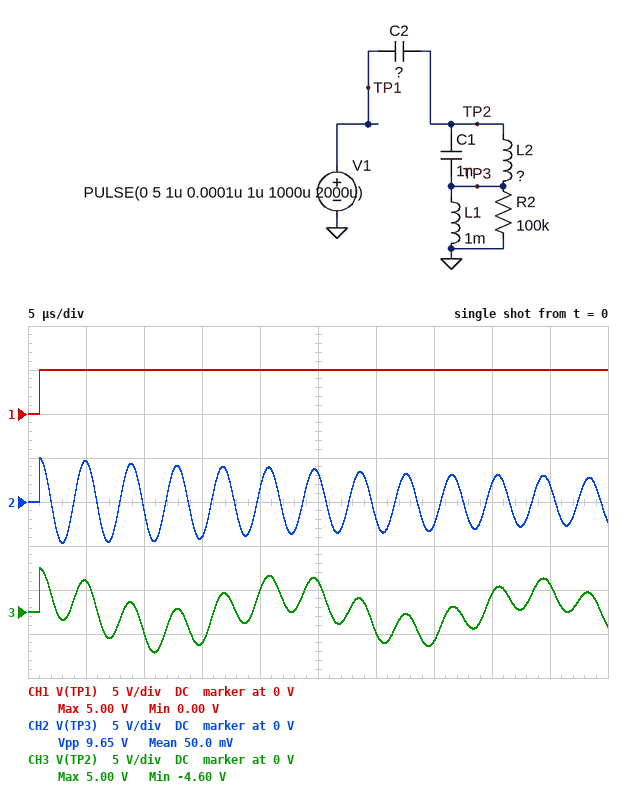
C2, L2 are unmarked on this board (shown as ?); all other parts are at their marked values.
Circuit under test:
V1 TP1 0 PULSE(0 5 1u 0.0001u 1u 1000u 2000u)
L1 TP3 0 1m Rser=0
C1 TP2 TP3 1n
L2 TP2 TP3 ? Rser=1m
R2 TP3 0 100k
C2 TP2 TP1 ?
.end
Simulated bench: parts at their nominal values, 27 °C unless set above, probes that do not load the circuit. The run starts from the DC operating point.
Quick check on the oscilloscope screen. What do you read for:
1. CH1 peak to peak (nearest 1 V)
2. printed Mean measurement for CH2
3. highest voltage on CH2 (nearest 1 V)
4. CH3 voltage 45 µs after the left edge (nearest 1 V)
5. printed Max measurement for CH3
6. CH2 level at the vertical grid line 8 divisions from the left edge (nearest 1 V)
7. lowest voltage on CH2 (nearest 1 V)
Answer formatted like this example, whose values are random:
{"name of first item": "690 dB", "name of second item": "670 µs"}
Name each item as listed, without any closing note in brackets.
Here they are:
{"CH1 peak to peak": "5 V", "printed Mean measurement for CH2": "50.0 mV", "highest voltage on CH2": "5 V", "CH3 voltage 45 µs after the left edge": "3 V", "printed Max measurement for CH3": "5.00 V", "CH2 level at the vertical grid line 8 divisions from the left edge": "2 V", "lowest voltage on CH2": "-5 V"}
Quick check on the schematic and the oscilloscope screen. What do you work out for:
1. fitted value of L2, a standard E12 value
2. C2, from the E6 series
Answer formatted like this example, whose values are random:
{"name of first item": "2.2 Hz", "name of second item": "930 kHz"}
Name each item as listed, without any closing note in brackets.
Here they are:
{"fitted value of L2, a standard E12 value": "6.8 mH", "C2, from the E6 series": "680 pF"}
